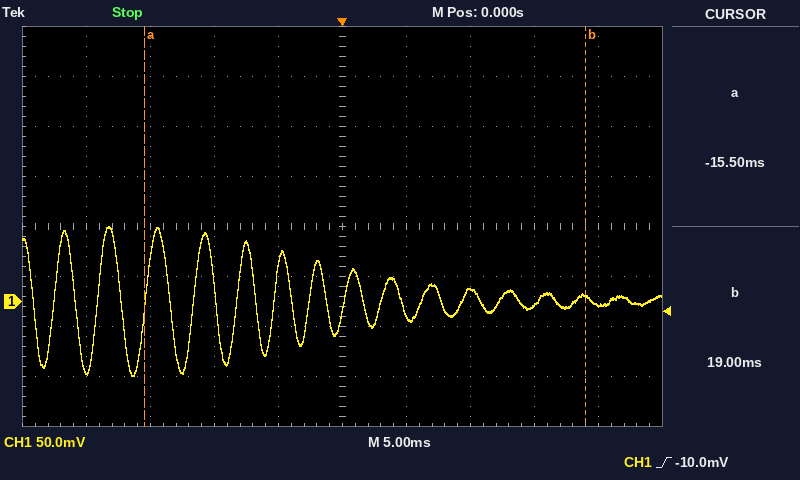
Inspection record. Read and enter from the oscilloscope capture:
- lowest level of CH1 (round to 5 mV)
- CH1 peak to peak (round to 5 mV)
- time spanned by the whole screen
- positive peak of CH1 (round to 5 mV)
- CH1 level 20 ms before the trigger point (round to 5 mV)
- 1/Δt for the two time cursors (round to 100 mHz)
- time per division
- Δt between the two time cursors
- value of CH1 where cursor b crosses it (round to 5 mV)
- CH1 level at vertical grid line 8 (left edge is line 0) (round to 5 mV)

-75 mV
150 mV
50 ms
75 mV
-70 mV
29.0 Hz
5 ms
34.5 ms
5 mV
-5 mV
